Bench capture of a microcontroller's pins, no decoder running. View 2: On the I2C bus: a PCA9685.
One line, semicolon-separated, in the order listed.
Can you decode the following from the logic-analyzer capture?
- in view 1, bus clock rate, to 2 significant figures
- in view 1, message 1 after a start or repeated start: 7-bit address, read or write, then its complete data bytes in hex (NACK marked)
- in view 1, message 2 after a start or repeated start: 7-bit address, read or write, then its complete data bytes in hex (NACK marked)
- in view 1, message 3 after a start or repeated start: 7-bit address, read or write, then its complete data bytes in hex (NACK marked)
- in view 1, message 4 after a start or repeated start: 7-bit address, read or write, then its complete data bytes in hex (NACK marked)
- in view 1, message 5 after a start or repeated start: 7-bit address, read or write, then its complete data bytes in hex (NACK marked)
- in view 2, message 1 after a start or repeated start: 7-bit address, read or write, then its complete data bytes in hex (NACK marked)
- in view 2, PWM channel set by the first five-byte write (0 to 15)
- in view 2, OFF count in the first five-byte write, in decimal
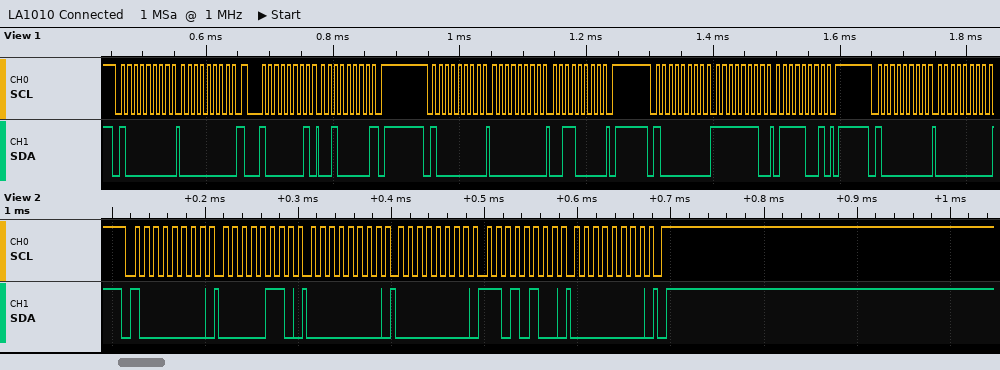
100 kHz; 0x40 write: 00; 0x40 read: 20 NACK; 0x40 write: 00 30; 0x40 write: FE 79; 0x40 write: 00; 0x40 write: 06 00 00 D4 00; 0; 212
